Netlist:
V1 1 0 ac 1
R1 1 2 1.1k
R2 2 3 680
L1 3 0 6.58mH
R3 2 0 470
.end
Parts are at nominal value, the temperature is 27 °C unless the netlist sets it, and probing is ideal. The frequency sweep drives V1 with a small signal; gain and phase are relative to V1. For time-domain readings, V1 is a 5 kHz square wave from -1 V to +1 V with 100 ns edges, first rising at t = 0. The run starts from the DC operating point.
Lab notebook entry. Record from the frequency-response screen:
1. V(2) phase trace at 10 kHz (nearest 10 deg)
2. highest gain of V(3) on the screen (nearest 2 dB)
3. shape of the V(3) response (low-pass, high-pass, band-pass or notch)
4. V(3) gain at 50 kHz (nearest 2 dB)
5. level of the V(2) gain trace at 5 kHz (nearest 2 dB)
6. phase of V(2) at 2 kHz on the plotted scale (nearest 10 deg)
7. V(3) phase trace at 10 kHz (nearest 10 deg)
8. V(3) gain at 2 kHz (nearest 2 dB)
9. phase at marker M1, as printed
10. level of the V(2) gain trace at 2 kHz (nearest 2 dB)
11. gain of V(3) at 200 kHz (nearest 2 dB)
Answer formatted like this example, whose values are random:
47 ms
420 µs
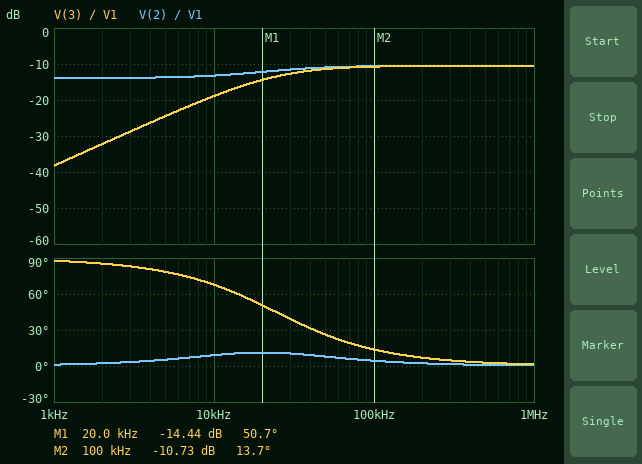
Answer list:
10 deg
-10 dB
high-pass
-12 dB
-14 dB
0 deg
70 deg
-32 dB
50.7 deg
-14 dB
-10 dB
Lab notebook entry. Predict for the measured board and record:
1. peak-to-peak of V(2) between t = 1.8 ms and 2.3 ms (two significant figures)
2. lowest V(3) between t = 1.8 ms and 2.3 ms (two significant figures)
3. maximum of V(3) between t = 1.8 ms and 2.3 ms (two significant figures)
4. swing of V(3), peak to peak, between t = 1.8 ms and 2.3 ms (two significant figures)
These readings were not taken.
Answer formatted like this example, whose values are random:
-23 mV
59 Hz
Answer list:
790 mV
-590 mV
590 mV
1.2 V
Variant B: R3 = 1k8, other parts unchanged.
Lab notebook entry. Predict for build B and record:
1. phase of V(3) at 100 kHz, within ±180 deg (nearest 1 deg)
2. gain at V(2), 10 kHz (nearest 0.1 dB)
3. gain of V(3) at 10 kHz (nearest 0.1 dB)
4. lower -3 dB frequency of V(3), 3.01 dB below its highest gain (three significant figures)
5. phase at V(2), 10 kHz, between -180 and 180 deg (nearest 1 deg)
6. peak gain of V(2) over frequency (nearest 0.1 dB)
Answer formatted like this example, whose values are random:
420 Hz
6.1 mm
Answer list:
18 deg
-9.2 dB
-14.9 dB
33.0 kHz
14 deg
-4.1 dB
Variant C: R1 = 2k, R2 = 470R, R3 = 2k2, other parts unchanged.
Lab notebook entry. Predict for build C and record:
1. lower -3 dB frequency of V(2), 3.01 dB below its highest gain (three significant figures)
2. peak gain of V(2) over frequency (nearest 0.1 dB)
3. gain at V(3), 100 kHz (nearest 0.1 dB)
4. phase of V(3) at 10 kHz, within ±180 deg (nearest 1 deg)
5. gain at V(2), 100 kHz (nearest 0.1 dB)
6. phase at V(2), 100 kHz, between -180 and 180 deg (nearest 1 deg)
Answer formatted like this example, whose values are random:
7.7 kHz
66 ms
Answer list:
33.0 kHz
-5.6 dB
-6.2 dB
75 deg
-6.1 dB
14 deg
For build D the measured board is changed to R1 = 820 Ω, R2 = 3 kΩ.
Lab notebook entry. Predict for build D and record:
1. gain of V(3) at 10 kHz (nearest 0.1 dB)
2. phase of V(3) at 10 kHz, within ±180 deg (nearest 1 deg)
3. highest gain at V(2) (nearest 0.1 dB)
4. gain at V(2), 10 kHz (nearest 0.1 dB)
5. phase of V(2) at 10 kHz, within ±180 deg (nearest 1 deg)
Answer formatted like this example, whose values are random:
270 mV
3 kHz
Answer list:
-26.9 dB
83 deg
-8.8 dB
-9.6 dB
1 deg
